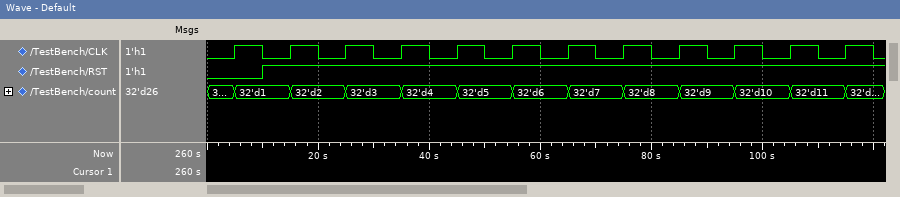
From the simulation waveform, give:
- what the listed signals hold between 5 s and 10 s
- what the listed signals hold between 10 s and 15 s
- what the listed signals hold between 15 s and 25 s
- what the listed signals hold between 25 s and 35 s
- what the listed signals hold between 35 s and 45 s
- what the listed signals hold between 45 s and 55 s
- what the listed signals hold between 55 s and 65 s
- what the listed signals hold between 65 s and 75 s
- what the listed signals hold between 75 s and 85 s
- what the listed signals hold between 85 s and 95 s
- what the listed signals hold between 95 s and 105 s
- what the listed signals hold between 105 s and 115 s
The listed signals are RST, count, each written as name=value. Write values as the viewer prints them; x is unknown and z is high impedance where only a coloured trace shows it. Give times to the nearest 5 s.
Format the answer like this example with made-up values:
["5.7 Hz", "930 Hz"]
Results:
["RST=0, count=32'd1", "RST=1, count=32'd1", "RST=1, count=32'd2", "RST=1, count=32'd3", "RST=1, count=32'd4", "RST=1, count=32'd5", "RST=1, count=32'd6", "RST=1, count=32'd7", "RST=1, count=32'd8", "RST=1, count=32'd9", "RST=1, count=32'd10", "RST=1, count=32'd11"]
